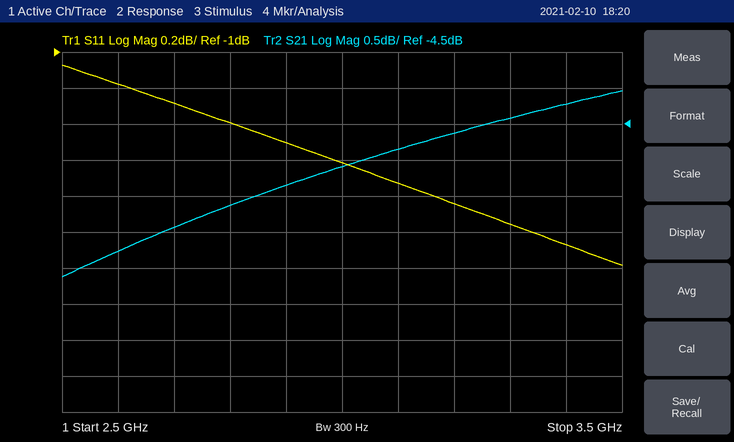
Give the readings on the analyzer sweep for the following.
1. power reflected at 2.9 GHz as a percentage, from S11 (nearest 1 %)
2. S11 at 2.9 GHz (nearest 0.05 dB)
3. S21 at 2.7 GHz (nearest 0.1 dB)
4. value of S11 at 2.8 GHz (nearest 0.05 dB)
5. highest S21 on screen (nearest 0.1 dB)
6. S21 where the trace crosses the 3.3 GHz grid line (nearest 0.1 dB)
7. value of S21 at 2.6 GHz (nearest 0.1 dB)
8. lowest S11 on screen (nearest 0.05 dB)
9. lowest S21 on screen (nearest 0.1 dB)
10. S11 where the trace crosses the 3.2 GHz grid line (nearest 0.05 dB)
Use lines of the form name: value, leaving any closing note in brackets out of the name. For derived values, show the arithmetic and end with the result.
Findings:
power reflected at 2.9 GHz as a percentage, from S11: 10^(-1.5/10) ≈ 71 %
S11 at 2.9 GHz: -1.50 dB
S21 at 2.7 GHz: -5.9 dB
value of S11 at 2.8 GHz: -1.40 dB
highest S21 on screen: -4.0 dB
S21 where the trace crosses the 3.3 GHz grid line: -4.4 dB
value of S21 at 2.6 GHz: -6.3 dB
lowest S11 on screen: -2.20 dB
lowest S21 on screen: -6.6 dB
S11 where the trace crosses the 3.2 GHz grid line: -1.85 dB
